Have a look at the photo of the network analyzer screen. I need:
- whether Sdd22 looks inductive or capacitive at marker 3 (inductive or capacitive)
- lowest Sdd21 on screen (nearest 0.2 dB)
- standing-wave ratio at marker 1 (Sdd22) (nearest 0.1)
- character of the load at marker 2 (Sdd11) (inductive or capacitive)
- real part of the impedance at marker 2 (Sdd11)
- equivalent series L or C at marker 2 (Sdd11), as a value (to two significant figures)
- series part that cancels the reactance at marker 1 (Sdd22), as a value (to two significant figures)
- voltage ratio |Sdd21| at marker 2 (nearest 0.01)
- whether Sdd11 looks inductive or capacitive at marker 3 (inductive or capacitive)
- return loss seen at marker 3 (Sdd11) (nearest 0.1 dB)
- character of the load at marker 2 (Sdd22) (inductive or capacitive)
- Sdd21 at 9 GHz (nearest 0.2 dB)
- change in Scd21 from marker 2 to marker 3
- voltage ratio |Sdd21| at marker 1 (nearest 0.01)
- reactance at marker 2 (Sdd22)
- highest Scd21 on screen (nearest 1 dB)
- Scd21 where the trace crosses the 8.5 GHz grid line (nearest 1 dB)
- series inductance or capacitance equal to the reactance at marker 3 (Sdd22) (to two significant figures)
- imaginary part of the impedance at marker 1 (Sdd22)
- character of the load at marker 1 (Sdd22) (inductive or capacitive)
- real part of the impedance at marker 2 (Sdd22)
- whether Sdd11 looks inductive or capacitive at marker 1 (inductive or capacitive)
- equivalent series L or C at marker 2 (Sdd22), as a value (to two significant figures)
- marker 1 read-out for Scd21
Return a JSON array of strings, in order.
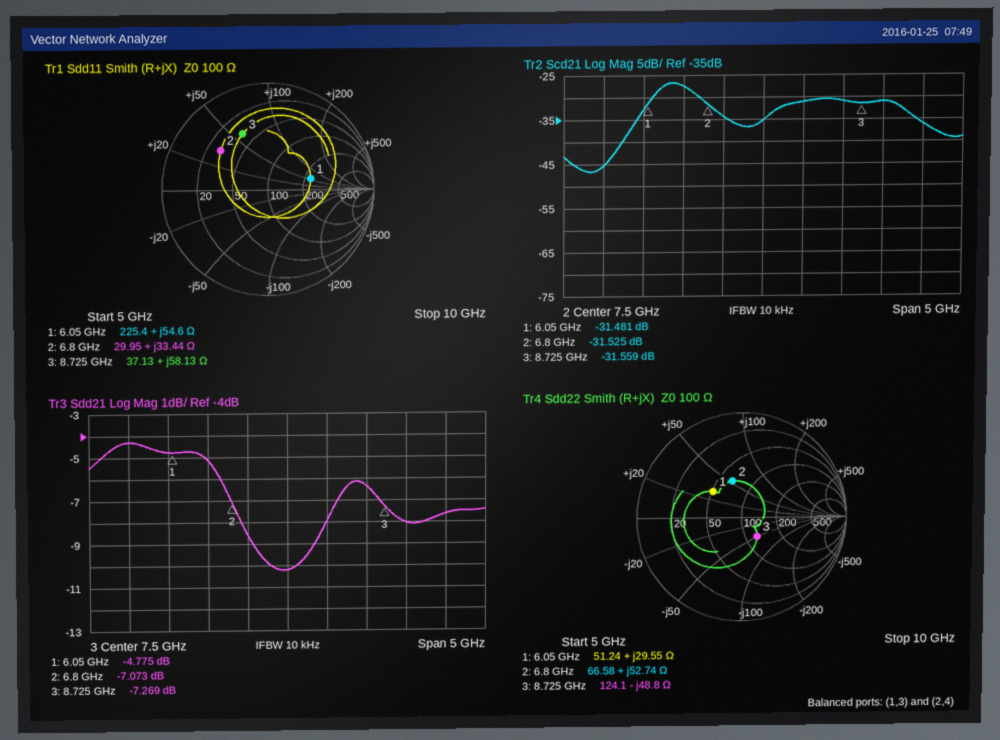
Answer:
["capacitive", "-10.2 dB", "2.2", "inductive", "29.95 Ω", "780 pH", "890 fF", "0.44", "inductive", "4.8 dB", "inductive", "-8.0 dB", "-0.034 dB", "0.58", "+52.74 Ω", "-27 dB", "-31 dB", "370 fF", "+29.55 Ω", "inductive", "66.58 Ω", "inductive", "1.2 nH", "-31.481 dB"]
